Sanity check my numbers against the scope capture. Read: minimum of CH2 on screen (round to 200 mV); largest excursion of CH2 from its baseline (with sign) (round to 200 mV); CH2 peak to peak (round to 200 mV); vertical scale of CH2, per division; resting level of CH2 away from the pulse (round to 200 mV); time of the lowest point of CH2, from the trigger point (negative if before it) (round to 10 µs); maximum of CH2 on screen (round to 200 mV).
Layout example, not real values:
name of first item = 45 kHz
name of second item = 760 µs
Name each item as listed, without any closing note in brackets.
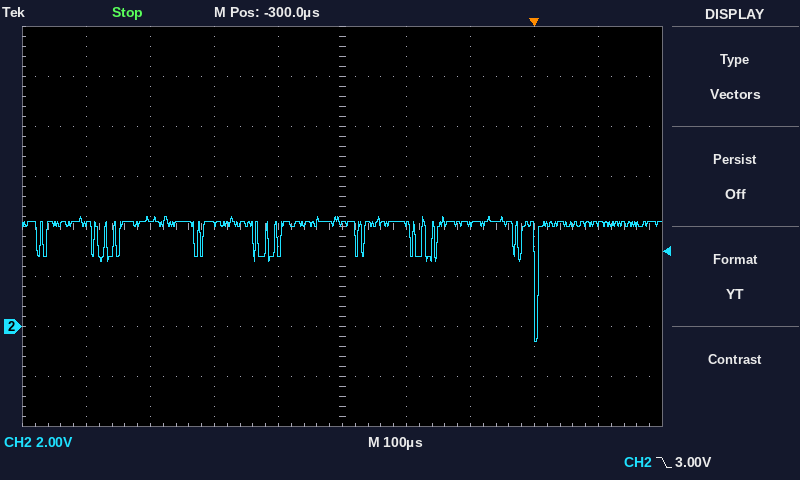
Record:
minimum of CH2 on screen = -600 mV
largest excursion of CH2 from its baseline (with sign) = -4.8 V
CH2 peak to peak = 5.0 V
vertical scale of CH2, per division = 2 V
resting level of CH2 away from the pulse = 4.2 V
time of the lowest point of CH2, from the trigger point (negative if before it) = 0 µs
maximum of CH2 on screen = 4.4 V
